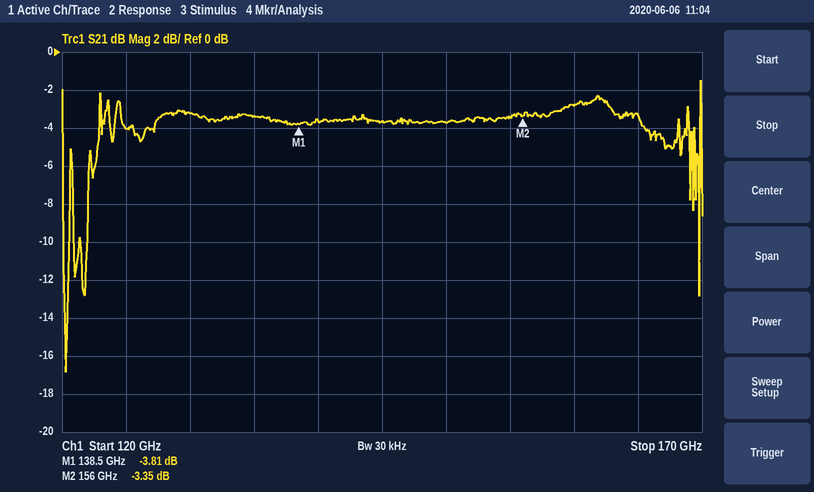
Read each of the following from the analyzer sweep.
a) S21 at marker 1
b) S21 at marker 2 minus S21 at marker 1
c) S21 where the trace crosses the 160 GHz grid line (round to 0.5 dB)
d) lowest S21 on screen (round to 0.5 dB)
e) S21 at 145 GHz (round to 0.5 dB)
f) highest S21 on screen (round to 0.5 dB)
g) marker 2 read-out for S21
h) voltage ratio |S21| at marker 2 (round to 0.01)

-3.81 dB
0.46 dB
-3.0 dB
-17.0 dB
-3.5 dB
-1.5 dB
-3.35 dB
0.68
